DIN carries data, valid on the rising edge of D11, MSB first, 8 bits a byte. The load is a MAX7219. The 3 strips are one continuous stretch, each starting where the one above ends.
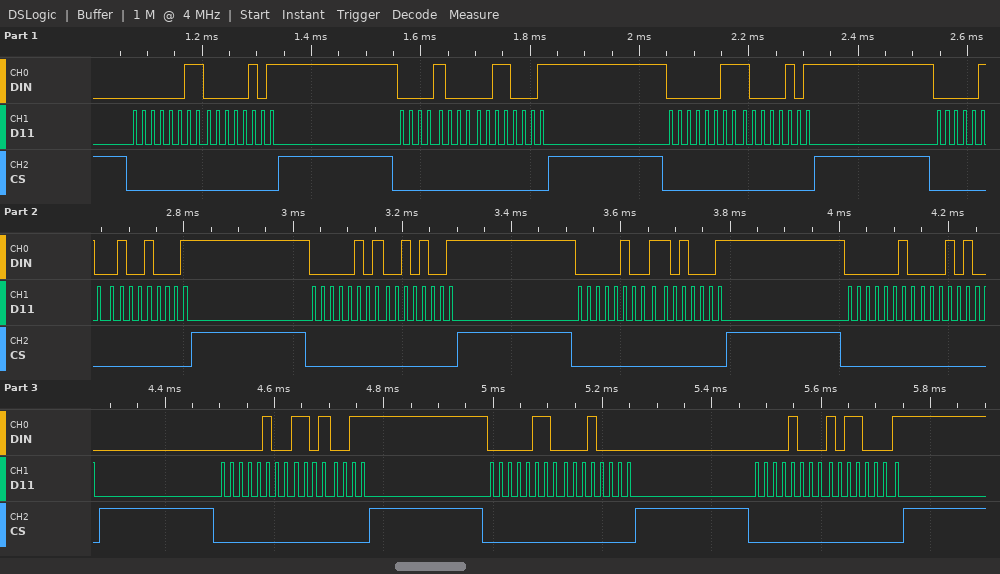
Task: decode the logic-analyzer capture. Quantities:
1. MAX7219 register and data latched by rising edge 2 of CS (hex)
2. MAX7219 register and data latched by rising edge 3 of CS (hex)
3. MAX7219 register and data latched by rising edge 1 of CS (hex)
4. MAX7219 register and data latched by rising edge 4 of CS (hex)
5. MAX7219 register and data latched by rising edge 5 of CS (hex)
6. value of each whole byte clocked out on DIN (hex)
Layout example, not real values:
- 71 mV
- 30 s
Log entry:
- register 0x8, data 0x31
- register 0x3, data 0x85
- register 0x3, data 0x05
- register 0x4, data 0x91
- register 0x5, data 0x29
- 03 05 08 31 03 85 04 91 05 29 04 D1 02 14 04 D3 06 10 08 B1
